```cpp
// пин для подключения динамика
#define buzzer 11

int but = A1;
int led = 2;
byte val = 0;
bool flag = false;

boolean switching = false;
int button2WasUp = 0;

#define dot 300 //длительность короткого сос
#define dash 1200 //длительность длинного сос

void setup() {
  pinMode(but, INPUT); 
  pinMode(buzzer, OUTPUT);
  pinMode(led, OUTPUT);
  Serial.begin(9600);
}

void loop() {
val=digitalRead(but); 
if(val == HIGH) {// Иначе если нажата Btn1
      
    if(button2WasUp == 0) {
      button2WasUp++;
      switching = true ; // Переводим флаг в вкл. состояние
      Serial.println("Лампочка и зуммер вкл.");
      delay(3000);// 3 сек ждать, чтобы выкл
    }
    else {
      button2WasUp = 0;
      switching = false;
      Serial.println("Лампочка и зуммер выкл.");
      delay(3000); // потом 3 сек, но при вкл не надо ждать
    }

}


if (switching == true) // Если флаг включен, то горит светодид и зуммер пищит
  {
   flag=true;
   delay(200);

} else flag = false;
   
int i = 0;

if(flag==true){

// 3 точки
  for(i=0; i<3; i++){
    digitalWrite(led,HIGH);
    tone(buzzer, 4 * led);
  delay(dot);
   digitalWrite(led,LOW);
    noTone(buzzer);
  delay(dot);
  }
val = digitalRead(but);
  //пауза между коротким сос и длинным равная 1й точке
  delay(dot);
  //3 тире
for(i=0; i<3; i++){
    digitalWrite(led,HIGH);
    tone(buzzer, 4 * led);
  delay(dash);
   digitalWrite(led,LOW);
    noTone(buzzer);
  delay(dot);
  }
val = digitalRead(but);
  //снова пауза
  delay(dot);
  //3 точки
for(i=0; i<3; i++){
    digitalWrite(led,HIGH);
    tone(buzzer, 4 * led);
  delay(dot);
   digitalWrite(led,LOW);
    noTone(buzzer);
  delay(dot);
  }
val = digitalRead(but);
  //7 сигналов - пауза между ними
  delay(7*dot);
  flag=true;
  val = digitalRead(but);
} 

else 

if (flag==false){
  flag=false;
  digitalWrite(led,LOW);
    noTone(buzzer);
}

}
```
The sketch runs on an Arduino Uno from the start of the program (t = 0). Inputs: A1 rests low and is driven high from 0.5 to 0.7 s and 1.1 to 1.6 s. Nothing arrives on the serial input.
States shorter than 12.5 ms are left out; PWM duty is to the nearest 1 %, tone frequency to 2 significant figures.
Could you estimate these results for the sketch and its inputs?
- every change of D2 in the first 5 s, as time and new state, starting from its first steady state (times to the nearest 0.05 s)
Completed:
0 s low; 3.7 s high; 4 s low; 4.3 s high; 4.6 s low; 4.9 s high
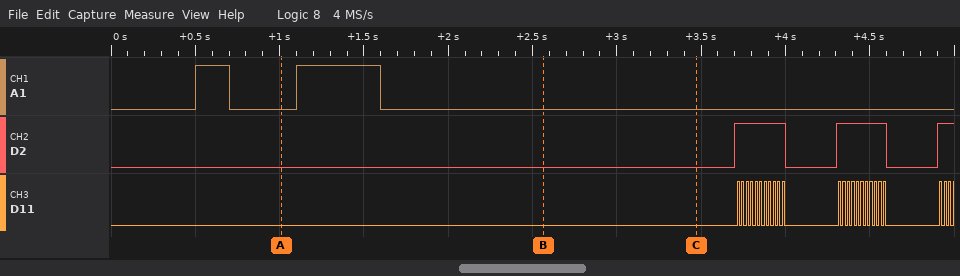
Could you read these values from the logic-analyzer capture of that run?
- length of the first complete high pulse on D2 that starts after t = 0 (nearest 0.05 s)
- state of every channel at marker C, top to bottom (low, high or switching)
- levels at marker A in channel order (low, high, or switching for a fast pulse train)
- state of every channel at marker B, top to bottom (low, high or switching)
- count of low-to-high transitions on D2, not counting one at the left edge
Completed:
0.30 s
A1 low, D2 low, D11 low
A1 low, D2 low, D11 low
A1 low, D2 low, D11 low
3
